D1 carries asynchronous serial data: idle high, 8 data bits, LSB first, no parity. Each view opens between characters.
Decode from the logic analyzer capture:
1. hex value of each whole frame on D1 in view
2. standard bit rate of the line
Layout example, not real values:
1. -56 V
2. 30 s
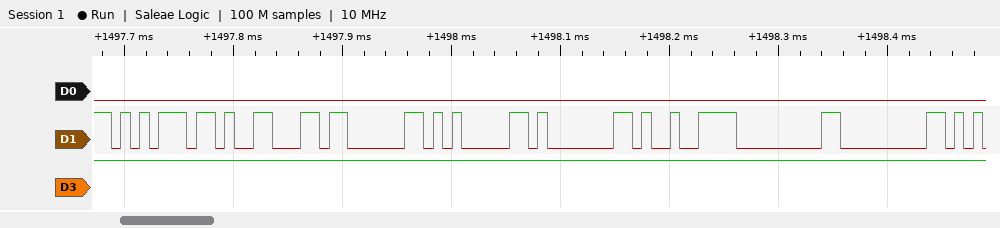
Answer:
1. 75, 19, 03, 05, 01, C9, 00, 00
2. 115200 baud
